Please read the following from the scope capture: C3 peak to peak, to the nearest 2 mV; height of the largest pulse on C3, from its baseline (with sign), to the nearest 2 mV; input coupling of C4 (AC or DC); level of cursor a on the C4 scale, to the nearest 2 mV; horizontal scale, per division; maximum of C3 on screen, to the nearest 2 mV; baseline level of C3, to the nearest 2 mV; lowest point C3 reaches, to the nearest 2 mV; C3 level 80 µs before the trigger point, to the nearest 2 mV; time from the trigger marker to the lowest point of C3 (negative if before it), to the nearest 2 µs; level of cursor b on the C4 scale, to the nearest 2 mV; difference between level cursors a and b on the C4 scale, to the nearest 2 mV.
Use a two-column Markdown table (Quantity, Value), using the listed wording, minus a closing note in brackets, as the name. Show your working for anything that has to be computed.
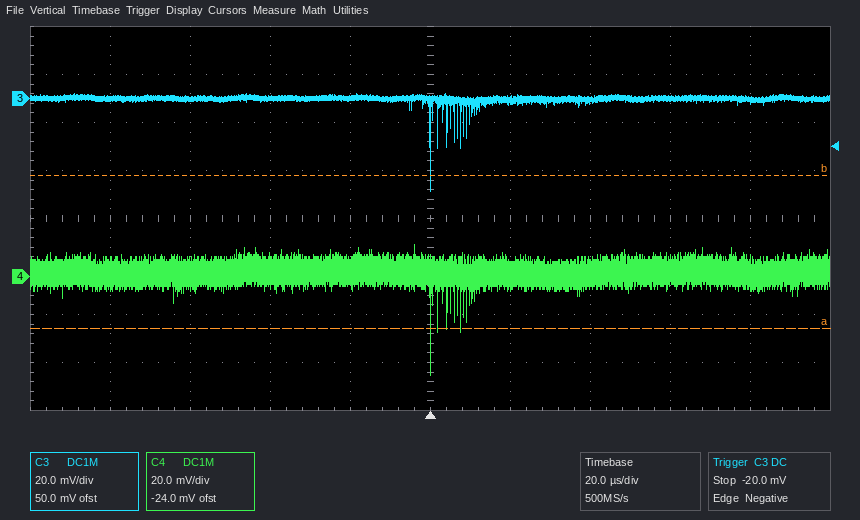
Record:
| Quantity | Value |
|---|---|
| C3 peak to peak, to the nearest 2 mV | 2 mV − (-38 mV) = 40 mV |
| height of the largest pulse on C3, from its baseline (with sign), to the nearest 2 mV | -38 mV − (0 mV) = -38 mV |
| input coupling of C4 | DC |
| level of cursor a on the C4 scale, to the nearest 2 mV | -22 mV |
| horizontal scale, per division | 20 µs |
| maximum of C3 on screen, to the nearest 2 mV | 2 mV |
| baseline level of C3, to the nearest 2 mV | 0 mV |
| lowest point C3 reaches, to the nearest 2 mV | -38 mV |
| C3 level 80 µs before the trigger point, to the nearest 2 mV | 0 mV |
| time from the trigger marker to the lowest point of C3 (negative if before it), to the nearest 2 µs | 0 µs |
| level of cursor b on the C4 scale, to the nearest 2 mV | 42 mV |
| difference between level cursors a and b on the C4 scale, to the nearest 2 mV | 64 mV |
